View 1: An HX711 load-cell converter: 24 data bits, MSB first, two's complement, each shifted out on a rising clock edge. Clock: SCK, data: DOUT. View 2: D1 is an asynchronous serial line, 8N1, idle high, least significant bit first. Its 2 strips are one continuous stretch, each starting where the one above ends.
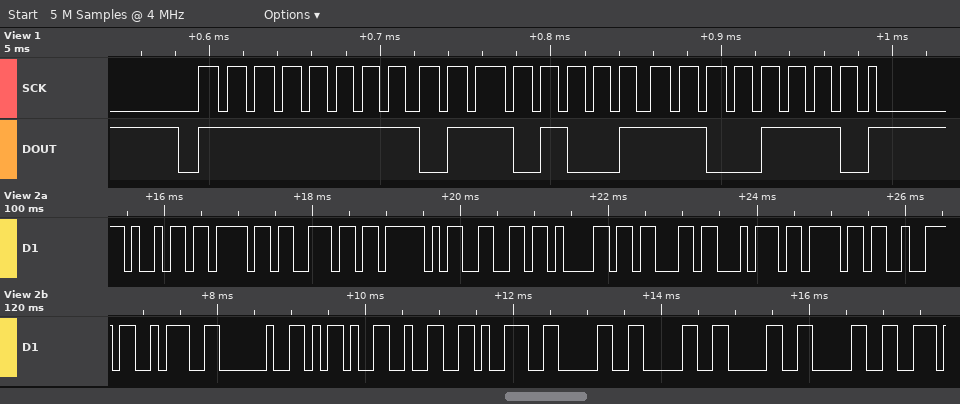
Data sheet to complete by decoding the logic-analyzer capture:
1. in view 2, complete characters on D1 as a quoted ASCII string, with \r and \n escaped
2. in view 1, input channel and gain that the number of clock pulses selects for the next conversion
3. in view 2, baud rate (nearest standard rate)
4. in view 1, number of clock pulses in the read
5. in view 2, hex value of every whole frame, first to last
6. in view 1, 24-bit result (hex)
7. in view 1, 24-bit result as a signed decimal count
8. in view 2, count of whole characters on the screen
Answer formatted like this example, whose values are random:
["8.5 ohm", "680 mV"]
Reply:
["\"ion_factor: -290000\"", "channel A, gain 128", "9600 baud", "25", "69 6F 6E 5F 66 61 63 74 6F 72 3A 20 2D 32 39 30 30 30 30", "0xFF69CE", "-38450", "19"]
